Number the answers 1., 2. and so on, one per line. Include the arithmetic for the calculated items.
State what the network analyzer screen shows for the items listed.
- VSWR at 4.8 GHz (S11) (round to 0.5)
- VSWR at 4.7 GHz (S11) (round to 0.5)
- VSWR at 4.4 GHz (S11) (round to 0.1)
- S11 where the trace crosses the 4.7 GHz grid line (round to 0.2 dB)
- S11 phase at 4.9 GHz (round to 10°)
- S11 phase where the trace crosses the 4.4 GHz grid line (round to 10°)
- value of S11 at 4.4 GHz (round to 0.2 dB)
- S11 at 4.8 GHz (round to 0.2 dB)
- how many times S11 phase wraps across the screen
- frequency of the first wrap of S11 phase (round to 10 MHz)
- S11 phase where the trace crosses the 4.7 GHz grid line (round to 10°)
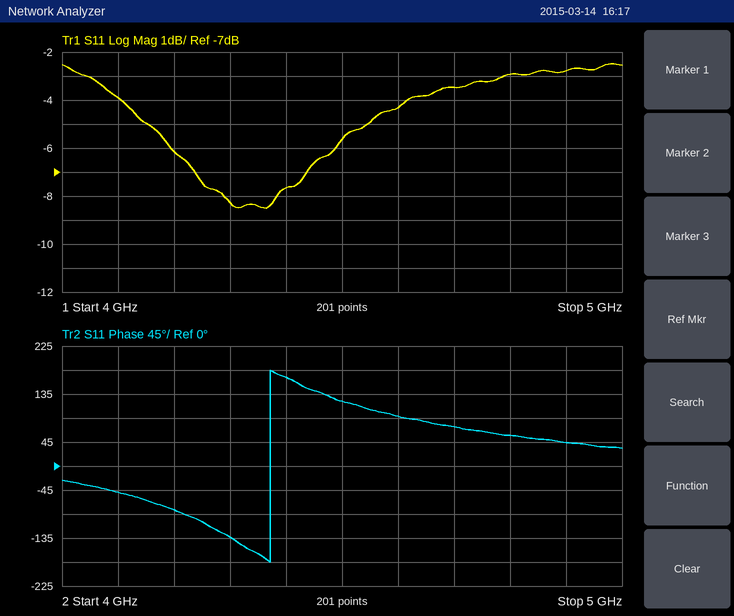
1. |Γ| = 10^(-3/20) = 0.7079; VSWR = (1 + 0.7079)/(1 − 0.7079) ≈ 5.85, so 6.0 to the nearest 0.5
2. |Γ| = 10^(-3.4/20) = 0.6761; VSWR = (1 + 0.6761)/(1 − 0.6761) ≈ 5.17, so 5.0 to the nearest 0.5
3. |Γ| = 10^(-7.6/20) = 0.4169; VSWR = (1 + 0.4169)/(1 − 0.4169) ≈ 2.4
4. -3.4 dB
5. 40°
6. 170°
7. -7.6 dB
8. -3.0 dB
9. 1
10. 4.37 GHz
11. 70°
